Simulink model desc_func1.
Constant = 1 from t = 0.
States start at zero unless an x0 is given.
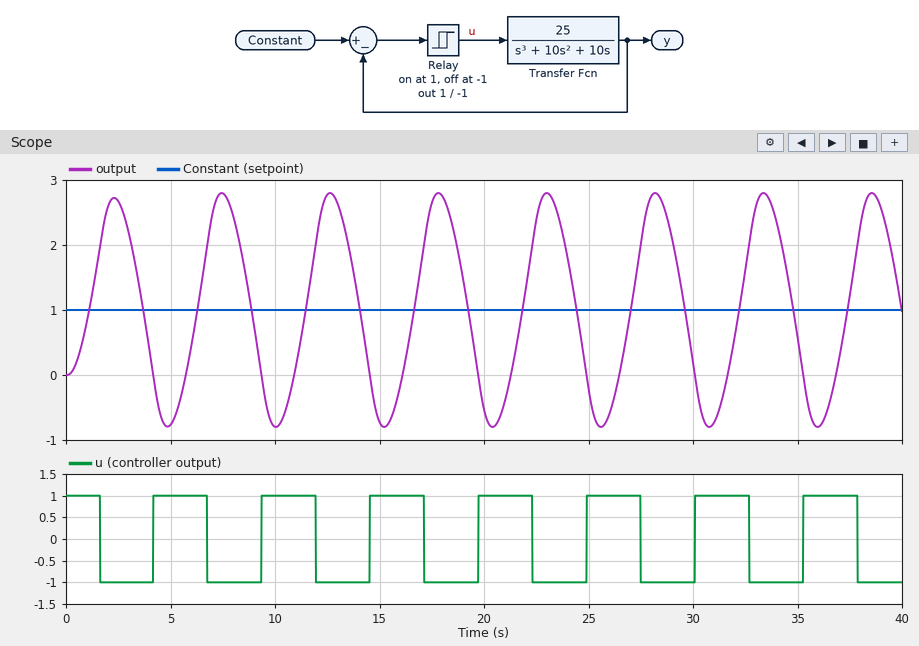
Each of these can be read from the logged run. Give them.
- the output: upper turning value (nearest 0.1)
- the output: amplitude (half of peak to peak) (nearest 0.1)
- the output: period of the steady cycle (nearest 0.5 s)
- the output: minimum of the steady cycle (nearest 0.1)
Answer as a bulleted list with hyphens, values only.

- 2.8
- 1.8
- 5.0 s
- -0.8
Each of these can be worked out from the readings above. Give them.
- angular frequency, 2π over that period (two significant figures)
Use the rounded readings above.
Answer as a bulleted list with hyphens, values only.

- 1.3 rad/s
